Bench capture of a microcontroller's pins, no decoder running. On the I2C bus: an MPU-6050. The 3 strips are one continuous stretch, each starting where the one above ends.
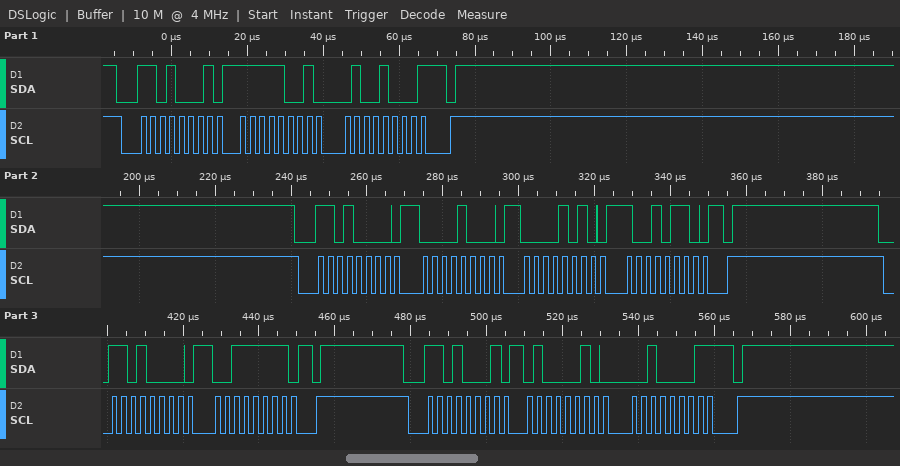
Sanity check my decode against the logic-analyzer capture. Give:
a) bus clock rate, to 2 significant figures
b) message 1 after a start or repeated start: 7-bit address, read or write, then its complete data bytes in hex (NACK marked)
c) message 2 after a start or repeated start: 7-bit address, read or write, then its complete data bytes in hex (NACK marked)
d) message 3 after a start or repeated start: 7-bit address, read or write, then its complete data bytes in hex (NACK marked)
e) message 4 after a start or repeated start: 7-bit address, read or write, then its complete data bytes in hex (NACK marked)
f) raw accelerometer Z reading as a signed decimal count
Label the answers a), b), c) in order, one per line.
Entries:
a) 400 kHz
b) 0x68 read: F9 48 NACK
c) 0x68 write: 08 0A 96
d) 0x68 write: 3F
e) 0x68 read: 42 21 NACK
f) 16929
